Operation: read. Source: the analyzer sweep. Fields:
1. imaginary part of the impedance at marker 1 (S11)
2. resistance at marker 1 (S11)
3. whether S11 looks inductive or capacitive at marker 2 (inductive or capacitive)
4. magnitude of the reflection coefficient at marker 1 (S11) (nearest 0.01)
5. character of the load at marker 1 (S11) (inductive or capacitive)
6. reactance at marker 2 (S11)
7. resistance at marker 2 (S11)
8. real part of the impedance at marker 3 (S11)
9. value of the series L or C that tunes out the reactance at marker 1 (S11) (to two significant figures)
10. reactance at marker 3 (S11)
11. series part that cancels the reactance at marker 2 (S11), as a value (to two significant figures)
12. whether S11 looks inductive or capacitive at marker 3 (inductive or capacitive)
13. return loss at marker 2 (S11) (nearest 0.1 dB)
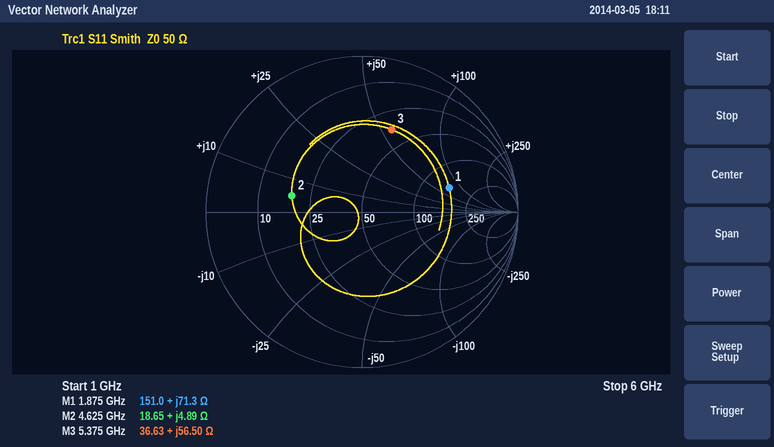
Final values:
+71.3 Ω
151.0 Ω
inductive
0.58
inductive
+4.89 Ω
18.65 Ω
36.63 Ω
1.2 pF
+56.50 Ω
7.0 pF
inductive
6.7 dB
